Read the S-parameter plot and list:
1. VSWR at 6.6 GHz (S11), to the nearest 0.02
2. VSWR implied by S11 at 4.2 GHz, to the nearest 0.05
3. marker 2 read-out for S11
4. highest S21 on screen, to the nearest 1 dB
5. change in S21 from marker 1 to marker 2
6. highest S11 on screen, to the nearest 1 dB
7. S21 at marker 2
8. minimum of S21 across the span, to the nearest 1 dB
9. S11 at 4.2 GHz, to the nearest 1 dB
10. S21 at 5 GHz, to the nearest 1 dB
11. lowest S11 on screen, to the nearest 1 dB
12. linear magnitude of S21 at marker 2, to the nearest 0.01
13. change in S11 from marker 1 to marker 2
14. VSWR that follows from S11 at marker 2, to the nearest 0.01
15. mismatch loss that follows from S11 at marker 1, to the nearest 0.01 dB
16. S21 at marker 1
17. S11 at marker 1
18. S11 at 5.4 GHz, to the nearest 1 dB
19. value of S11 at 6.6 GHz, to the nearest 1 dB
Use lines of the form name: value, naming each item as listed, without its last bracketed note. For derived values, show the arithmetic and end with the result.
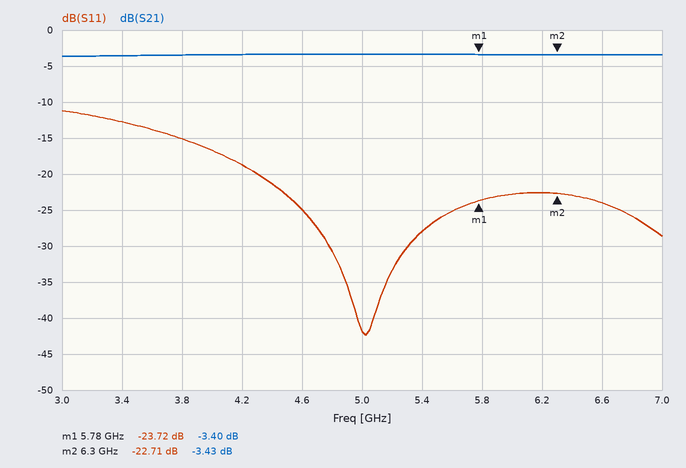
VSWR at 6.6 GHz (S11), to the nearest 0.02: |Γ| = 10^(-24/20) = 0.0631; VSWR = (1 + 0.0631)/(1 − 0.0631) ≈ 1.13, so 1.14 to the nearest 0.02
VSWR implied by S11 at 4.2 GHz, to the nearest 0.05: |Γ| = 10^(-19/20) = 0.1122; VSWR = (1 + 0.1122)/(1 − 0.1122) ≈ 1.25
marker 2 read-out for S11: -22.71 dB
highest S21 on screen, to the nearest 1 dB: -3 dB
change in S21 from marker 1 to marker 2: -3.43 − (-3.4) = -0.03 dB
highest S11 on screen, to the nearest 1 dB: -11 dB
S21 at marker 2: -3.43 dB
minimum of S21 across the span, to the nearest 1 dB: -4 dB
S11 at 4.2 GHz, to the nearest 1 dB: -19 dB
S21 at 5 GHz, to the nearest 1 dB: -3 dB
lowest S11 on screen, to the nearest 1 dB: -42 dB
linear magnitude of S21 at marker 2, to the nearest 0.01: 10^(-3.43/20) ≈ 0.67
change in S11 from marker 1 to marker 2: -22.71 − (-23.72) = 1.01 dB
VSWR that follows from S11 at marker 2, to the nearest 0.01: (1 + 0.0732)/(1 − 0.0732) ≈ 1.16
mismatch loss that follows from S11 at marker 1, to the nearest 0.01 dB: −10 log10(1 − 10^(-23.72/10)) ≈ 0.02 dB
S21 at marker 1: -3.40 dB
S11 at marker 1: -23.72 dB
S11 at 5.4 GHz, to the nearest 1 dB: -28 dB
value of S11 at 6.6 GHz, to the nearest 1 dB: -24 dB
